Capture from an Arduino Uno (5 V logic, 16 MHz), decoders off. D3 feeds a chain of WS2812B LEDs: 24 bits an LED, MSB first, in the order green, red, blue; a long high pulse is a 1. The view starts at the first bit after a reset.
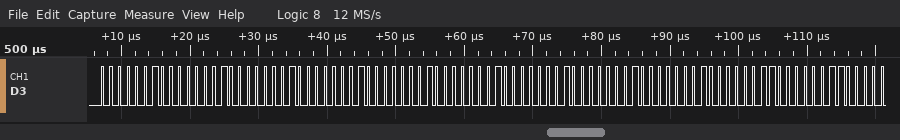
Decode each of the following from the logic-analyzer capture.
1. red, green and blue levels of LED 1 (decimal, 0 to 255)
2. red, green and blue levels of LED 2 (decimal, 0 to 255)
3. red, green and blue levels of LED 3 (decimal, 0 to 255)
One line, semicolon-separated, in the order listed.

2, 2, 2; 2, 2, 2; 2, 2, 2
